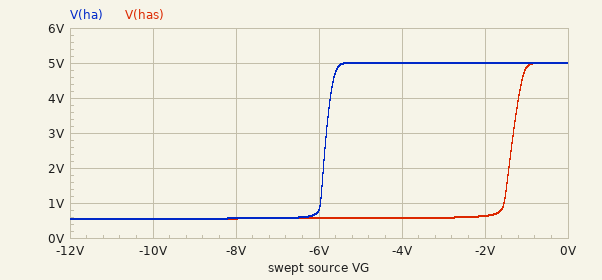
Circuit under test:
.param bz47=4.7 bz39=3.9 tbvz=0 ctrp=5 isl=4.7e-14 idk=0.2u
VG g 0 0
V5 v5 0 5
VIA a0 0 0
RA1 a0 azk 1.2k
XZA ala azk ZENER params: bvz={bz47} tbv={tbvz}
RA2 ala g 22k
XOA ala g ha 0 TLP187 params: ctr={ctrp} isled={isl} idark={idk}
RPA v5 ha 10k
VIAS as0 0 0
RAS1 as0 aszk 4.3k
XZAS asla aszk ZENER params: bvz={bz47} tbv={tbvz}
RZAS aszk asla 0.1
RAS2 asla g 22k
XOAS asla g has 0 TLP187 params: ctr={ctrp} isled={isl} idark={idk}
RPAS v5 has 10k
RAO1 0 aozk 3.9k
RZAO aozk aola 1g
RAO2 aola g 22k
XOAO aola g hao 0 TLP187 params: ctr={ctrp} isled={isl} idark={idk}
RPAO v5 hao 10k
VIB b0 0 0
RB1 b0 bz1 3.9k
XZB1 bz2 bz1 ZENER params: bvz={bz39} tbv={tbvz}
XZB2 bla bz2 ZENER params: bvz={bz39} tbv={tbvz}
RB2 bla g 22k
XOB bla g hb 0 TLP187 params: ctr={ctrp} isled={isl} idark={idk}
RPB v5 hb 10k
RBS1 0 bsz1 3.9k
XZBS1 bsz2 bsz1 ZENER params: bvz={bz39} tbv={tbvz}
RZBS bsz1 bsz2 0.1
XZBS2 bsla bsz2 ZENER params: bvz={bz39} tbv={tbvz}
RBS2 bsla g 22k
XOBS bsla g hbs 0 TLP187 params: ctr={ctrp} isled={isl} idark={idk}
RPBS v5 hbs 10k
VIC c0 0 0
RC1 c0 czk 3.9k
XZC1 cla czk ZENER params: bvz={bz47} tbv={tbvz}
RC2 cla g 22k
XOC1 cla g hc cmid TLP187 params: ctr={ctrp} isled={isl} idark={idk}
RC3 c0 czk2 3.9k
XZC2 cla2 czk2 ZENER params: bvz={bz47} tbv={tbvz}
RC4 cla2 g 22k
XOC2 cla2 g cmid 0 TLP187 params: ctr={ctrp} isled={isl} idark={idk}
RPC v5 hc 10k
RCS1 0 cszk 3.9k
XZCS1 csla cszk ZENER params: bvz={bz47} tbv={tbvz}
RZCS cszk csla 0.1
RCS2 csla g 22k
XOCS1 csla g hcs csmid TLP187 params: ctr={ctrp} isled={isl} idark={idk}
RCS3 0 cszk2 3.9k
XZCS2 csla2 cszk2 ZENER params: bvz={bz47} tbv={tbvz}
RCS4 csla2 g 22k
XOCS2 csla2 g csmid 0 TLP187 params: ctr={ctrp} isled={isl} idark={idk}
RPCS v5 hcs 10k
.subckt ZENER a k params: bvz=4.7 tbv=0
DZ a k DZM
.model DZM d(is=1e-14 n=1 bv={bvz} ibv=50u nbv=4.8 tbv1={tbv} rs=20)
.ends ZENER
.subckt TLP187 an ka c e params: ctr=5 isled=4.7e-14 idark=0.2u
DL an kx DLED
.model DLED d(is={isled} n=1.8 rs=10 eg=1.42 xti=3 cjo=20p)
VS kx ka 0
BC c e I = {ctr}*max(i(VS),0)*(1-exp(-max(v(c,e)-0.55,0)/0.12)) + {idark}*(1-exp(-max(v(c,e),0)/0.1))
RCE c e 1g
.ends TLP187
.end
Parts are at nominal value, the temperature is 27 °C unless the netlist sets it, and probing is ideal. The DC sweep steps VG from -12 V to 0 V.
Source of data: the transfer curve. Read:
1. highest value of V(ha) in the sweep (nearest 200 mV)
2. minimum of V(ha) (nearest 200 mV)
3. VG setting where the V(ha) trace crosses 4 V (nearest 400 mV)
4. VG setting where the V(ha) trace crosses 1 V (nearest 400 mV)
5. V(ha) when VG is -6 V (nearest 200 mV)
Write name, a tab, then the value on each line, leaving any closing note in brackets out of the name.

highest value of V(ha) in the sweep	5.0 V
minimum of V(ha)	600 mV
VG setting where the V(ha) trace crosses 4 V	-5.6 V
VG setting where the V(ha) trace crosses 1 V	-6.0 V
V(ha) when VG is -6 V	800 mV
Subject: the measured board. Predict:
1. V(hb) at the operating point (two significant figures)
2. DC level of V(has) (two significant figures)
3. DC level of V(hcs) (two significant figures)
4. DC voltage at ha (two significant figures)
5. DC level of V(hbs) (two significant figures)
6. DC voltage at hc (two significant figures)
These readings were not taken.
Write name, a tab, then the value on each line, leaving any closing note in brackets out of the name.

V(hb) at the operating point	5.0 V
DC level of V(has)	5.0 V
DC level of V(hcs)	5.0 V
DC voltage at ha	5.0 V
DC level of V(hbs)	5.0 V
DC voltage at hc	5.0 V
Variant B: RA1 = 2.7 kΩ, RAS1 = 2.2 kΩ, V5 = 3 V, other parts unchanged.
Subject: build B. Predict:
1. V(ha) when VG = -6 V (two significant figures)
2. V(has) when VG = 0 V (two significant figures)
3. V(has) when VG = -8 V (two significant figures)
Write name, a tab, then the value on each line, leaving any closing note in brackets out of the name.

V(ha) when VG = -6 V	810 mV
V(has) when VG = 0 V	3.0 V
V(has) when VG = -8 V	550 mV
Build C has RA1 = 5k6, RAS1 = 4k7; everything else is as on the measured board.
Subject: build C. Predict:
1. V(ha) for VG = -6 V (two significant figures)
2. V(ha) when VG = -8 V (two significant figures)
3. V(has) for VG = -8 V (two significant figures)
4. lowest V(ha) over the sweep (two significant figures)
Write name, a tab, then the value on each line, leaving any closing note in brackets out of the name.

V(ha) for VG = -6 V	4.0 V
V(ha) when VG = -8 V	590 mV
V(has) for VG = -8 V	560 mV
lowest V(ha) over the sweep	560 mV
